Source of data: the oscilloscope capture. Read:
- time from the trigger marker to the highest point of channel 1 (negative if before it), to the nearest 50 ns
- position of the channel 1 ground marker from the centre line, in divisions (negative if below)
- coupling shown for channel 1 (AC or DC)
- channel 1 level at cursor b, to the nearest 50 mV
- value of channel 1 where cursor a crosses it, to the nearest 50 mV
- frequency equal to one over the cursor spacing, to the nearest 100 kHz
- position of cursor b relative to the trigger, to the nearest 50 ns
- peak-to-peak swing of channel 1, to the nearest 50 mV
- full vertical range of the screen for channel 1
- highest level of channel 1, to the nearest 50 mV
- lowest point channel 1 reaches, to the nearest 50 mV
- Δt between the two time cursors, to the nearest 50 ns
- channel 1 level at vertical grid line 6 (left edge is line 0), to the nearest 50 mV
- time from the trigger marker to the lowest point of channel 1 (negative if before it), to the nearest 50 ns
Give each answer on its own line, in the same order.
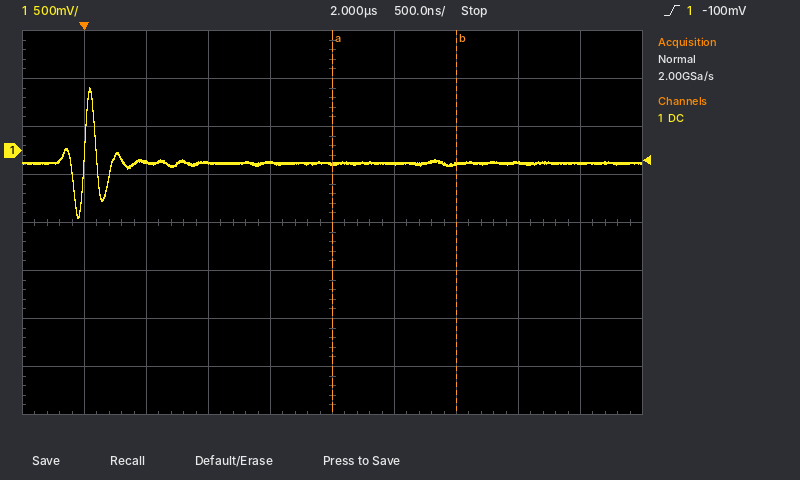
+50 ns
+1.5 div
DC
-150 mV
-150 mV
1.0 MHz
+3.00 µs
1.35 V
4 V
650 mV
-700 mV
1.00 µs
-150 mV
-50 ns
